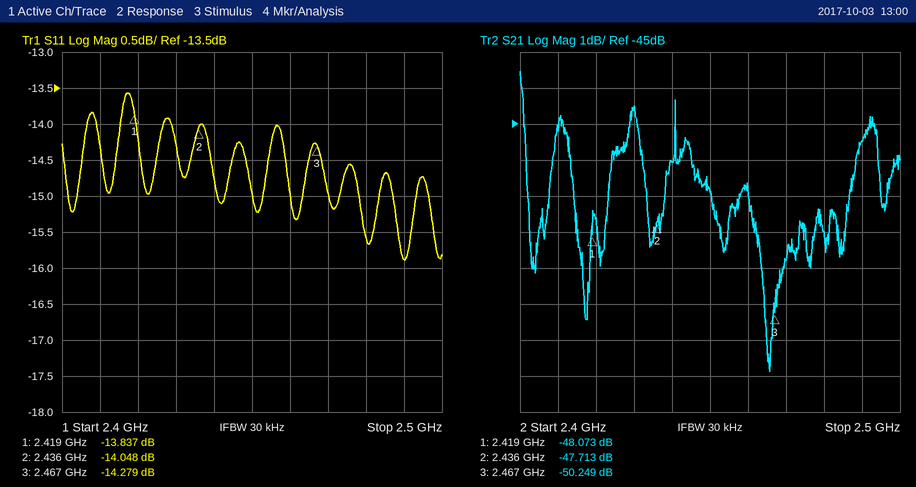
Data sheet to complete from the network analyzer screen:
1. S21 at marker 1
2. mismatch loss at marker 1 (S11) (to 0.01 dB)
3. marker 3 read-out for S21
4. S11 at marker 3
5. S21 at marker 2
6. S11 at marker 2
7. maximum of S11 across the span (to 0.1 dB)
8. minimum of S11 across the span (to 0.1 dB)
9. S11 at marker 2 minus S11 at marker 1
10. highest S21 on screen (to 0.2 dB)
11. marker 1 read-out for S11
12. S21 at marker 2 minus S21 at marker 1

-48.073 dB
0.18 dB
-50.249 dB
-14.279 dB
-47.713 dB
-14.048 dB
-13.6 dB
-15.9 dB
-0.211 dB
-43.6 dB
-13.837 dB
0.360 dB
